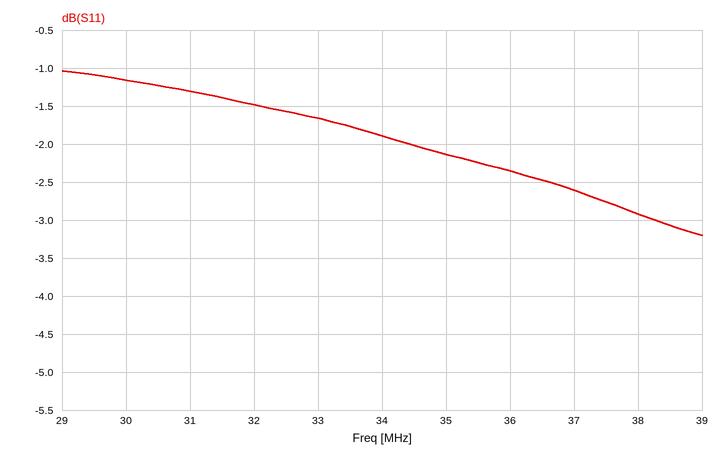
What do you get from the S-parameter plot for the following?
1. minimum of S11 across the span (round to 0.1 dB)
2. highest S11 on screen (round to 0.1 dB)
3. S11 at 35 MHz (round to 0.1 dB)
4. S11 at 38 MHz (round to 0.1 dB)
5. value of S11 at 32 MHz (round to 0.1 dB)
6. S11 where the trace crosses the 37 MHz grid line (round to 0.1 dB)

-3.2 dB
-1.0 dB
-2.1 dB
-2.9 dB
-1.5 dB
-2.6 dB
